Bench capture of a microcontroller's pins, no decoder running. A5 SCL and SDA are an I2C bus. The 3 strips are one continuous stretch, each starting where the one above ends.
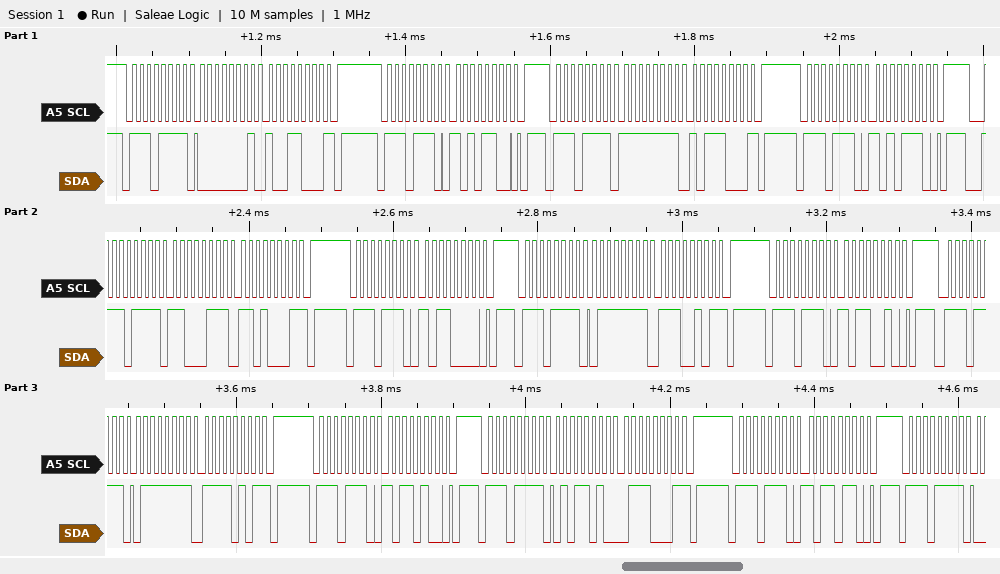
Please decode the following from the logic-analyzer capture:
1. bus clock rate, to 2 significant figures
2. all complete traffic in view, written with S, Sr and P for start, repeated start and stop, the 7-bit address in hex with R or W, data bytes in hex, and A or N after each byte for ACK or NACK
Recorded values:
100 kHz
S 77R A 01 A 98 N P S 77W A AC A P S 77R A FF A B8 N P S 77W A AE A P S 77R A C7 A D1 N P S 77W A B0 A P S 77R A 7F A E5 N P S 77W A B2 A P S 77R A 7F A F5 N P S 77W A B4 A P S 77R A 5A A 71 N P S 77W A B6 A P S 77R A
